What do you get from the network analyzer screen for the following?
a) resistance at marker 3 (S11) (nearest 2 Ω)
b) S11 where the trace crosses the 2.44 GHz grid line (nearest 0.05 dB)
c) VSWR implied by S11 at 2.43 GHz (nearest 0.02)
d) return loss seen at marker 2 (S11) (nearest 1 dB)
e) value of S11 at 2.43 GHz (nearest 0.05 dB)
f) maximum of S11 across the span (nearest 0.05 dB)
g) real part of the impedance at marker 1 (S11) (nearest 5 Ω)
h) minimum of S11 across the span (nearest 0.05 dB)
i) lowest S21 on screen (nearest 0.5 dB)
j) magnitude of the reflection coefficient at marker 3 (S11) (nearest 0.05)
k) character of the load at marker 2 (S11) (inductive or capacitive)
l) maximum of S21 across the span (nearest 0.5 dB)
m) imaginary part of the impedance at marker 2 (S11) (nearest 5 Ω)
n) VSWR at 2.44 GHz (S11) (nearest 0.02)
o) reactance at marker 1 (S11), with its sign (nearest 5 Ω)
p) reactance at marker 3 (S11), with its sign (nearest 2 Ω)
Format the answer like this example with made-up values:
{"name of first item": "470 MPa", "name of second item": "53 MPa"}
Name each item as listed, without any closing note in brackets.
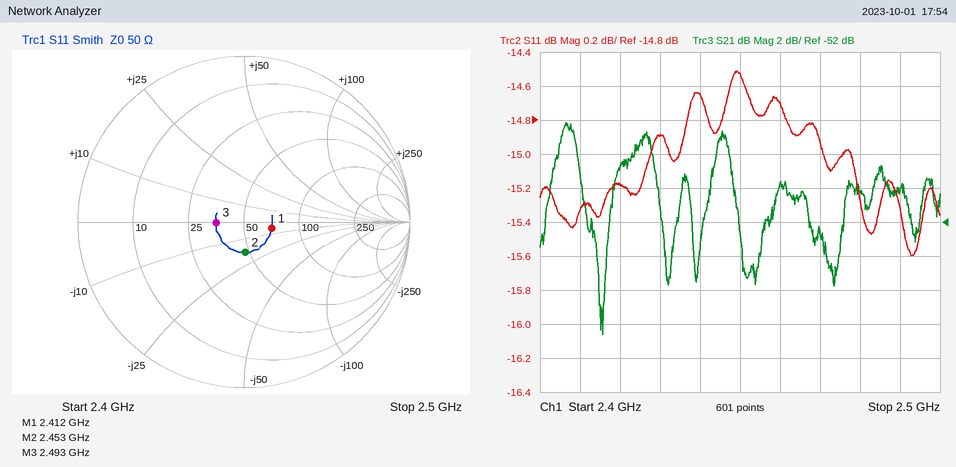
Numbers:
{"resistance at marker 3 (S11)": "36 Ω", "S11 where the trace crosses the 2.44 GHz grid line": "-14.65 dB", "VSWR implied by S11 at 2.43 GHz": "1.44", "return loss seen at marker 2 (S11)": "15 dB", "value of S11 at 2.43 GHz": "-14.90 dB", "maximum of S11 across the span": "-14.50 dB", "real part of the impedance at marker 1 (S11)": "70 Ω", "minimum of S11 across the span": "-15.60 dB", "lowest S21 on screen": "-58.5 dB", "magnitude of the reflection coefficient at marker 3 (S11)": "0.15", "character of the load at marker 2 (S11)": "capacitive", "maximum of S21 across the span": "-46.0 dB", "imaginary part of the impedance at marker 2 (S11)": "-20 Ω", "VSWR at 2.44 GHz (S11)": "1.46", "reactance at marker 1 (S11), with its sign": "-5 Ω", "reactance at marker 3 (S11), with its sign": "0 Ω"}
